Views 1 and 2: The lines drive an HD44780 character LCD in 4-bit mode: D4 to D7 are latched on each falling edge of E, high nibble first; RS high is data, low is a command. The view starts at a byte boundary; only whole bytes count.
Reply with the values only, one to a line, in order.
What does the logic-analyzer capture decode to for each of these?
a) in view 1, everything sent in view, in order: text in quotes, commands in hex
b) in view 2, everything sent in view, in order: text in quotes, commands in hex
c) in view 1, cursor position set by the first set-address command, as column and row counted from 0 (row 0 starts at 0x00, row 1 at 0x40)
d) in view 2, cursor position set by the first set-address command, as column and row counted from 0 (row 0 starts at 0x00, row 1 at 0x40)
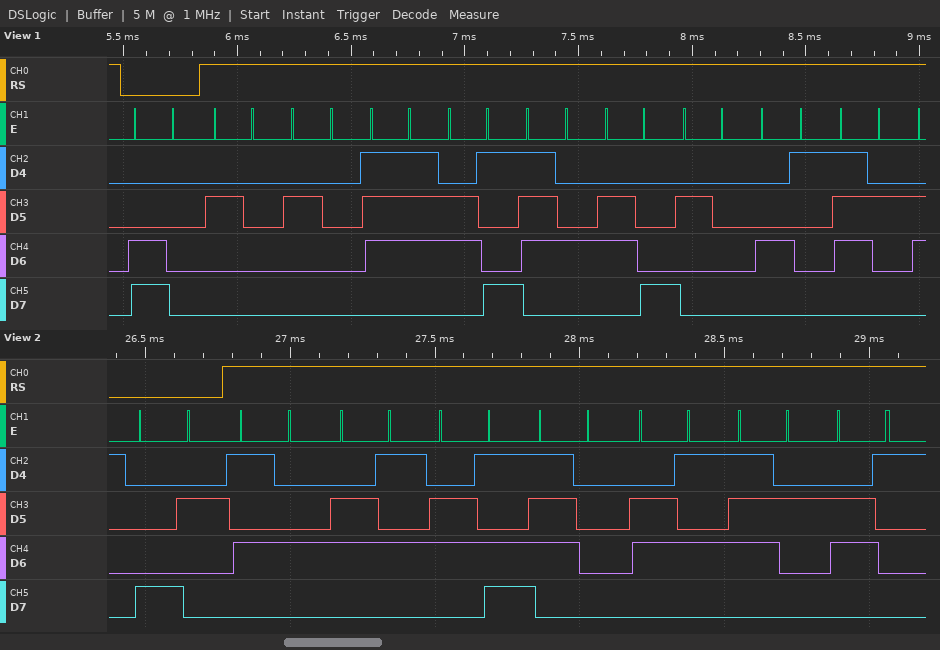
0xC0 "  with Ar"
0x82 "Tempera"
column 0, row 1
column 2, row 0
